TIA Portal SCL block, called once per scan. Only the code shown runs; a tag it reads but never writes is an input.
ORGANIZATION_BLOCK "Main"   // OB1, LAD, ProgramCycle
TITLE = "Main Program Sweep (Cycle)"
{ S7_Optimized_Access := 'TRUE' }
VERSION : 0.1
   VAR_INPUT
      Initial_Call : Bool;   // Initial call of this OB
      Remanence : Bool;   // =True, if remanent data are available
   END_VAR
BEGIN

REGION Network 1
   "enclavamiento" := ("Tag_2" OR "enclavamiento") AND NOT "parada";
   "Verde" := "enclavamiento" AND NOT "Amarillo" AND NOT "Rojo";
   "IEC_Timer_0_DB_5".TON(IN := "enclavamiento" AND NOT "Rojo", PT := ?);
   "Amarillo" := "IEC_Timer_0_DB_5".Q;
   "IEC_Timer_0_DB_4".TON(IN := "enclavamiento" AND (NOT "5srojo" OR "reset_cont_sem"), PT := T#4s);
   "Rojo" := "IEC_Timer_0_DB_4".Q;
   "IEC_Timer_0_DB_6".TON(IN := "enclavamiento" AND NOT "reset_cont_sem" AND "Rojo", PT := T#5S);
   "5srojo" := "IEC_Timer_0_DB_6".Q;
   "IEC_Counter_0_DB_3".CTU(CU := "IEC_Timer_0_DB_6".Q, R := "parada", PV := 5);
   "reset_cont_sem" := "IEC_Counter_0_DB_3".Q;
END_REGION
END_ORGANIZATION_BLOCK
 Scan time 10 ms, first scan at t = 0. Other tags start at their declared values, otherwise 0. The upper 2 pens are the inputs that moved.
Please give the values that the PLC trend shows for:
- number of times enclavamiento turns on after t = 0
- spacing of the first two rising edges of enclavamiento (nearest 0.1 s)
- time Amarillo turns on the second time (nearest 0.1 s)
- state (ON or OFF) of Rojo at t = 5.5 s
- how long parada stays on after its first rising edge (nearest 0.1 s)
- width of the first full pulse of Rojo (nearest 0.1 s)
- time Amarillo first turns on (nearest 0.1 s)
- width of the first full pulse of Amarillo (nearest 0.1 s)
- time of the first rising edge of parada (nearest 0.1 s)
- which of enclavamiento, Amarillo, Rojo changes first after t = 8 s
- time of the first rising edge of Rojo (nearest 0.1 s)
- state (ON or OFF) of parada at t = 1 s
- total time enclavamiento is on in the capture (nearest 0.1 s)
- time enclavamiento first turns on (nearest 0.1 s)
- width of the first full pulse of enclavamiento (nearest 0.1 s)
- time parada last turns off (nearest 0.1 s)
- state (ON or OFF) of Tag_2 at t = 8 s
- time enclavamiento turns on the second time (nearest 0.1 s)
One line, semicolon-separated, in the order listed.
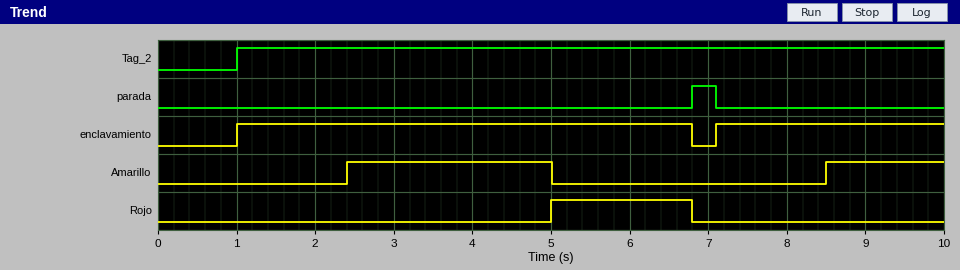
2; 6.1 s; 8.5 s; ON; 0.3 s; 1.8 s; 2.4 s; 2.6 s; 6.8 s; Amarillo; 5.0 s; OFF; 8.7 s; 1.0 s; 5.8 s; 7.1 s; ON; 7.1 s
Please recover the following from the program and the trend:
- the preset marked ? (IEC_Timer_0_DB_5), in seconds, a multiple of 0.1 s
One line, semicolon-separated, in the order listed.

1.4 s
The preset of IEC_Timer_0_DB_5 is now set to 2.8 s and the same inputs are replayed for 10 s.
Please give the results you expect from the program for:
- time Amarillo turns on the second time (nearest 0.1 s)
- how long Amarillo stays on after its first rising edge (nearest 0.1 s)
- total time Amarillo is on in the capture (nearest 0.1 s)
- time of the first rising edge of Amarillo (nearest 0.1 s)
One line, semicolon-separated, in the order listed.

9.9 s; 1.2 s; 1.3 s; 3.8 s
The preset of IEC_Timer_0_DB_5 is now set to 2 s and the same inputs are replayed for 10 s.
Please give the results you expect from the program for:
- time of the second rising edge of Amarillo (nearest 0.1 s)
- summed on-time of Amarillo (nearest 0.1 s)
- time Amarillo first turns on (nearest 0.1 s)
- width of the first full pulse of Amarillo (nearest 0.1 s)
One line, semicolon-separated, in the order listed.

9.1 s; 2.9 s; 3.0 s; 2.0 s
